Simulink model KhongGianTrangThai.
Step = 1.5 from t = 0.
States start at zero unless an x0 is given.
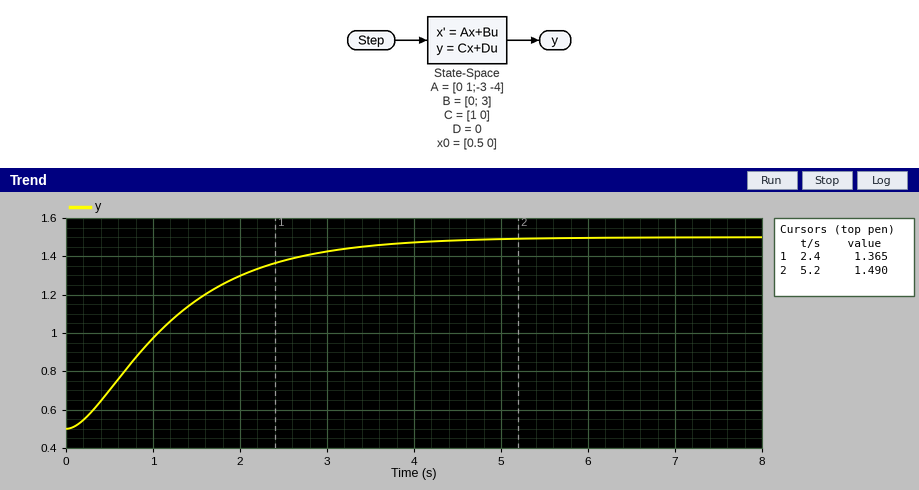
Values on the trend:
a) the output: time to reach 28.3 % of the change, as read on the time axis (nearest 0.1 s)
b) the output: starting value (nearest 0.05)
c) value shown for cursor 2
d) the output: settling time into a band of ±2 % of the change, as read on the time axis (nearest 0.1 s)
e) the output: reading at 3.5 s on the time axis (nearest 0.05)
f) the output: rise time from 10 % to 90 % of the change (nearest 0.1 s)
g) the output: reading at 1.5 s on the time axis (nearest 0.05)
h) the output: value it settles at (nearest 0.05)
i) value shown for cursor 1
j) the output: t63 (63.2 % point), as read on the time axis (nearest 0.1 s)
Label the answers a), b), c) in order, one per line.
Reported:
a) 0.6 s
b) 0.50
c) 1.490
d) 4.3 s
e) 1.45
f) 2.4 s
g) 1.15
h) 1.50
i) 1.365
j) 1.4 s
